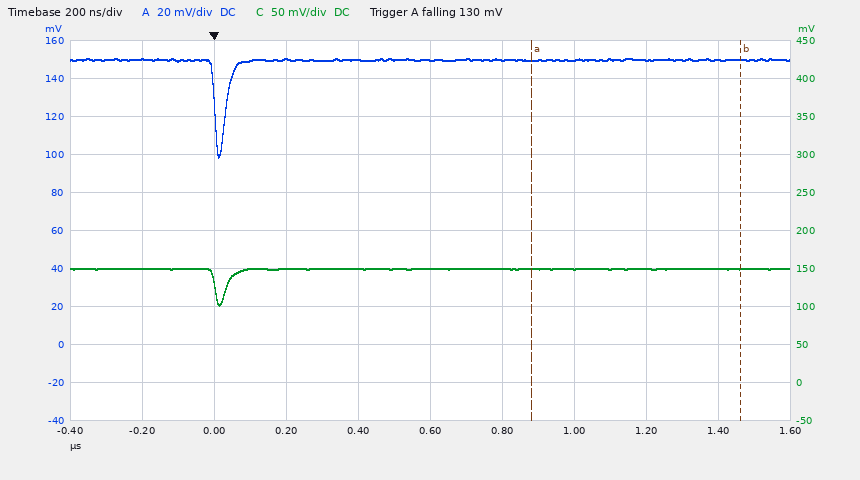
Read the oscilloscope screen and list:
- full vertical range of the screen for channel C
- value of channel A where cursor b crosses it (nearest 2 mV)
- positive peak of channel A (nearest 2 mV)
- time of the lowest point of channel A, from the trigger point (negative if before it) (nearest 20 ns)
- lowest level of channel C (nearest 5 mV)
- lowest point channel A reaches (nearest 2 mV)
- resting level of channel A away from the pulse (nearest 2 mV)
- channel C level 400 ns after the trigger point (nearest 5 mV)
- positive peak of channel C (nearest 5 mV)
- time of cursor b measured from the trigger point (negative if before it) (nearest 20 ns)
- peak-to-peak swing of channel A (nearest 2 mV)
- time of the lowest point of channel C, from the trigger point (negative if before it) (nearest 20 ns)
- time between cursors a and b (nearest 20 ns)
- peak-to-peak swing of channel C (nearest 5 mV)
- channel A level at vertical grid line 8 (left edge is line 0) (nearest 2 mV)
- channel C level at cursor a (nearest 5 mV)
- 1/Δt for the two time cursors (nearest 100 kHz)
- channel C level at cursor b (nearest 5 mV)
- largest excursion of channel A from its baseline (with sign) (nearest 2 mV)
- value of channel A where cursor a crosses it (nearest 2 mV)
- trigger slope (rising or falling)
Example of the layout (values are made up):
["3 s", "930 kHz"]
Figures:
["500 mV", "150 mV", "150 mV", "+20 ns", "100 mV", "98 mV", "150 mV", "150 mV", "150 mV", "+1.46 µs", "52 mV", "+20 ns", "580 ns", "50 mV", "150 mV", "150 mV", "1.7 MHz", "150 mV", "-52 mV", "150 mV", "falling"]
